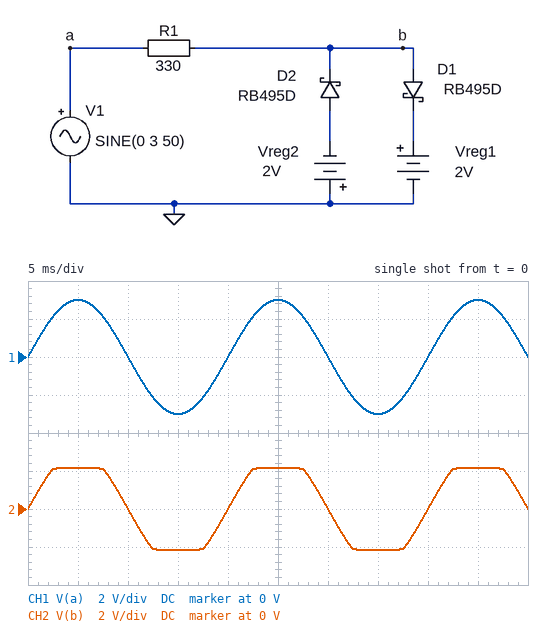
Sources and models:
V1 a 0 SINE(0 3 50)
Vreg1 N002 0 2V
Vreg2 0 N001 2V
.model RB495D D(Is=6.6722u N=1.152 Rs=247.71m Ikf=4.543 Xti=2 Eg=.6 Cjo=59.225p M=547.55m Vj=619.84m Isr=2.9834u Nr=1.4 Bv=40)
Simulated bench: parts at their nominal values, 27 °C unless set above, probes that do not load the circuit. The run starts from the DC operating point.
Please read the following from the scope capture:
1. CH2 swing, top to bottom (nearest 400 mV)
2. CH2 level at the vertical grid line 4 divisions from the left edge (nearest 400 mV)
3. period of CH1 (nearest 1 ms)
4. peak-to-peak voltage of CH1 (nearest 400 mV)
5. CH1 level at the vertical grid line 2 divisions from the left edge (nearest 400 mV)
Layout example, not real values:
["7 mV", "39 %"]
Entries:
["4.4 V", "0 V", "20 ms", "6.0 V", "0 V"]
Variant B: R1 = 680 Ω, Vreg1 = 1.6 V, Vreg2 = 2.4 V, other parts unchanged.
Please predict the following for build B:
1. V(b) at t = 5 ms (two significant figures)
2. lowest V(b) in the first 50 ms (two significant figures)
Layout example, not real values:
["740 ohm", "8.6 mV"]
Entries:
["1.8 V", "-2.5 V"]
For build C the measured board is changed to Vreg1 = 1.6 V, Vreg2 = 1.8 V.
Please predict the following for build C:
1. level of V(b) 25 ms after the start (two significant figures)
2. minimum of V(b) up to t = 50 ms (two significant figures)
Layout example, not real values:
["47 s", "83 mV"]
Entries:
["1.8 V", "-2.0 V"]
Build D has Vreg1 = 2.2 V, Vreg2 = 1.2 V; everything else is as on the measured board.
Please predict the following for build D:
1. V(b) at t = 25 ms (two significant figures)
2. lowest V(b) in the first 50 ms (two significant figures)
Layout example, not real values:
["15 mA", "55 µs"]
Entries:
["2.4 V", "-1.4 V"]
